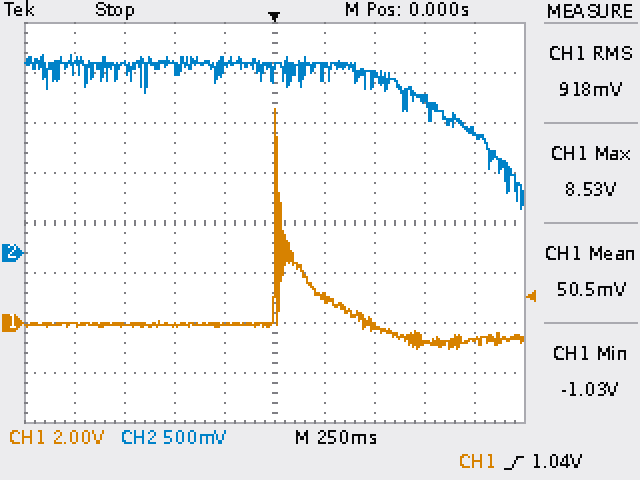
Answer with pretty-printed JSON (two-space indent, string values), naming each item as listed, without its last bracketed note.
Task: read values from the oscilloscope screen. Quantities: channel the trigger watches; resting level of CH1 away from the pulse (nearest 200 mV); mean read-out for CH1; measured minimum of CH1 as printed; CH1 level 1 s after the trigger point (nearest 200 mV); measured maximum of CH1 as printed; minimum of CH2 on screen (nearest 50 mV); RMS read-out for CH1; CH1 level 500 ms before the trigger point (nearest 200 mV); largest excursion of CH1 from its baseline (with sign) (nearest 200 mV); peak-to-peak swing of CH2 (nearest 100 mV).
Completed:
{
  "channel the trigger watches": "CH1",
  "resting level of CH1 away from the pulse": "0.0 V",
  "mean read-out for CH1": "50.5 mV",
  "measured minimum of CH1 as printed": "-1.03 V",
  "CH1 level 1 s after the trigger point": "-600 mV",
  "measured maximum of CH1 as printed": "8.53 V",
  "minimum of CH2 on screen": "450 mV",
  "RMS read-out for CH1": "918 mV",
  "CH1 level 500 ms before the trigger point": "0.0 V",
  "largest excursion of CH1 from its baseline (with sign)": "+8.6 V",
  "peak-to-peak swing of CH2": "1.50 V"
}
